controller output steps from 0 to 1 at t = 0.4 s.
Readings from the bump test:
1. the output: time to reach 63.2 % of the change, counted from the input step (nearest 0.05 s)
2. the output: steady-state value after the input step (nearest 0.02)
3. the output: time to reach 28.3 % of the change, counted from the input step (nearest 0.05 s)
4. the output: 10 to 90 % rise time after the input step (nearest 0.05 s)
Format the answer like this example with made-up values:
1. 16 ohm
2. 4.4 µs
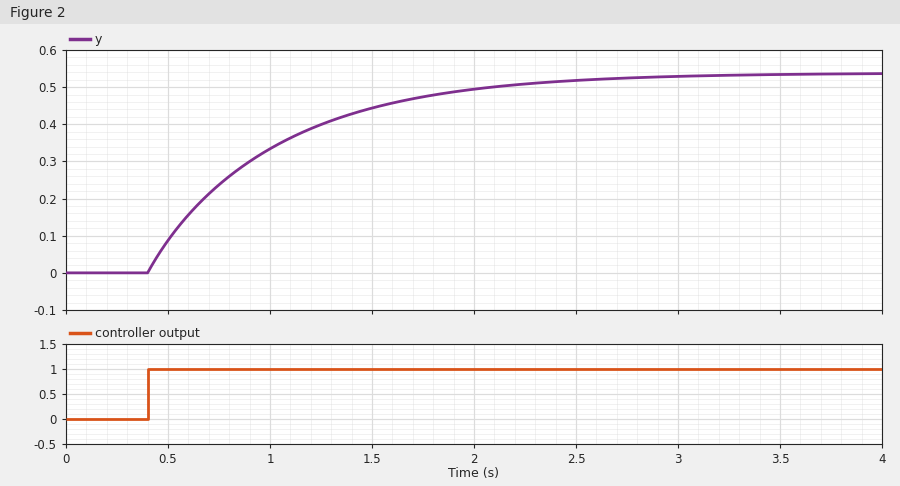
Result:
1. 0.60 s
2. 0.54
3. 0.20 s
4. 1.40 s
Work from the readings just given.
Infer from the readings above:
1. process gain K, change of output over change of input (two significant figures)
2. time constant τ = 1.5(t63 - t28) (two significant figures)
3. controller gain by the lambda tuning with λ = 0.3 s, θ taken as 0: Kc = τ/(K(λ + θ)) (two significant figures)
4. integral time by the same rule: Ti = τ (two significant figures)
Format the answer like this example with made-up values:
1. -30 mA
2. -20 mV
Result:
1. 0.54
2. 0.60 s
3. 3.7
4. 0.60 s
